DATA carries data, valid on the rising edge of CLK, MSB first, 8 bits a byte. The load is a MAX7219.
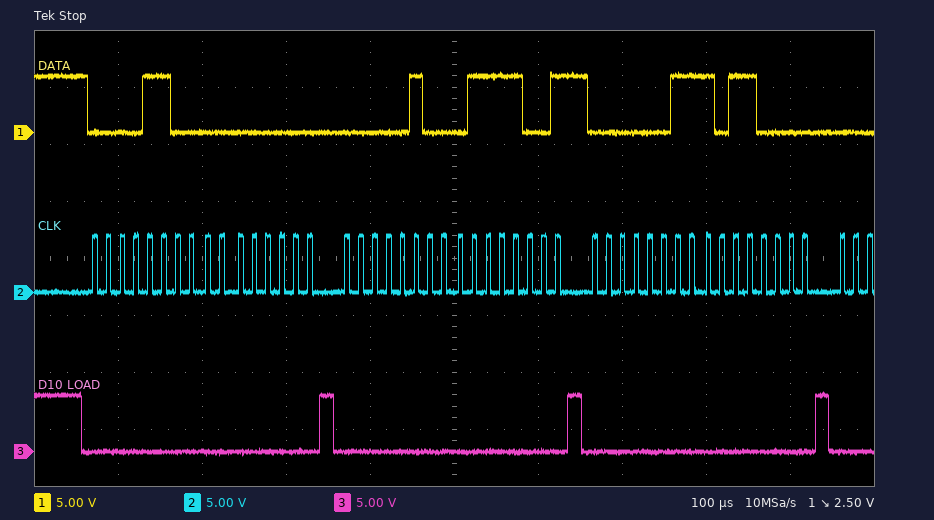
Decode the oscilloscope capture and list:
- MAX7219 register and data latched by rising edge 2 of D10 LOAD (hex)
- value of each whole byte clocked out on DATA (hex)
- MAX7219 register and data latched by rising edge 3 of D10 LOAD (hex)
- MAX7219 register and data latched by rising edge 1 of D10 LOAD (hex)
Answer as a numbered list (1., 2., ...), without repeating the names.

1. register 0x4, data 0x79
2. 0x0C 0x00 0x04 0x79 0x03 0xB0
3. register 0x3, data 0xB0
4. register 0xC, data 0x00
